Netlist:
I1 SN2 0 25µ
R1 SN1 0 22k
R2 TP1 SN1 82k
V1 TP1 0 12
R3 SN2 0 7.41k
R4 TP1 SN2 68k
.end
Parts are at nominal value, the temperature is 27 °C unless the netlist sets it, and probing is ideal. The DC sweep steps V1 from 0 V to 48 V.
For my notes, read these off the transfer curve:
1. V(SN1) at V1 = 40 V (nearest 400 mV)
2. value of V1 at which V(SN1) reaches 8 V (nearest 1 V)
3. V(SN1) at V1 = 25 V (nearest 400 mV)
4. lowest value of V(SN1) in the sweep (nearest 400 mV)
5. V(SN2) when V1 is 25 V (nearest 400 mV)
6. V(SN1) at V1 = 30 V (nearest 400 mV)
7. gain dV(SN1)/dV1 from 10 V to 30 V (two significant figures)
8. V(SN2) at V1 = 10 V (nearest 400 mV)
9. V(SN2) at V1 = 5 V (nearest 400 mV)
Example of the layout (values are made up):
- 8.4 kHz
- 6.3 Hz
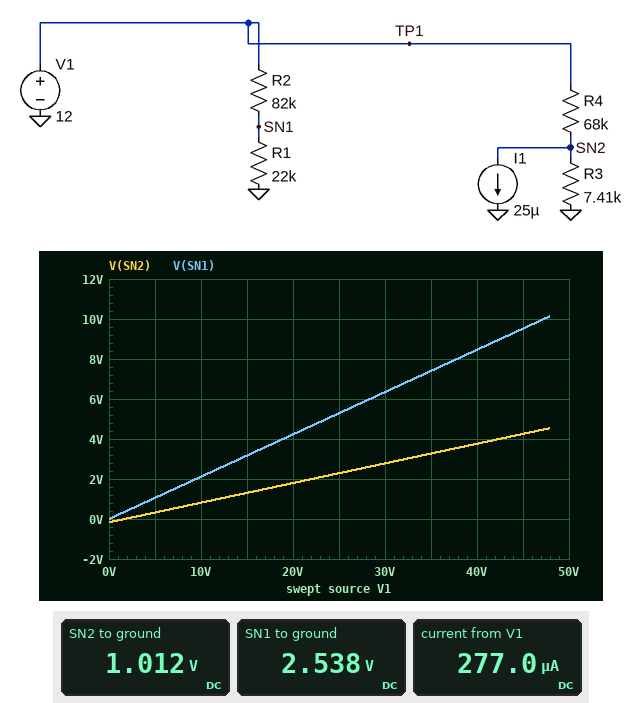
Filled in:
- 8.4 V
- 38 V
- 5.2 V
- 0 V
- 2.4 V
- 6.4 V
- 0.21 V/V
- 800 mV
- 400 mV
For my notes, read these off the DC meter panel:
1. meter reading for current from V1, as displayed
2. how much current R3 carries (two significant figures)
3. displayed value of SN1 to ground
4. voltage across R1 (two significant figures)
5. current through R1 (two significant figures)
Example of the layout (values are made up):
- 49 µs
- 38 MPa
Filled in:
- 277.0 µA
- 140 µA
- 2.538 V
- 2.5 V
- 120 µA
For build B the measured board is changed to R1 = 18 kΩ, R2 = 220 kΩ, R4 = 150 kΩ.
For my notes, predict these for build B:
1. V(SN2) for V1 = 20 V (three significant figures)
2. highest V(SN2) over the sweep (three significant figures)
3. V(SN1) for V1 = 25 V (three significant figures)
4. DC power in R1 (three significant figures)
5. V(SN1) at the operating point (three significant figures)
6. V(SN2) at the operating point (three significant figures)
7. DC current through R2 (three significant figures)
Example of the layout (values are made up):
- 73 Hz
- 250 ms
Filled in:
- 765 mV
- 2.08 V
- 1.89 V
- 45.8 µW
- 908 mV
- 388 mV
- 50.4 µA
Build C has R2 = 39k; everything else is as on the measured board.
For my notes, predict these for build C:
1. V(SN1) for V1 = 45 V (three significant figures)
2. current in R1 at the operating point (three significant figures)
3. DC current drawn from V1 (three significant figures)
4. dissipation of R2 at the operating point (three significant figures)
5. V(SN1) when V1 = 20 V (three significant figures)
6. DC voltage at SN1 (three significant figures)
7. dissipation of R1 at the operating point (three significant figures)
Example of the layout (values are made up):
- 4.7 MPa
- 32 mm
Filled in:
- 16.2 V
- 197 µA
- 358 µA
- 1.51 mW
- 7.21 V
- 4.33 V
- 851 µW
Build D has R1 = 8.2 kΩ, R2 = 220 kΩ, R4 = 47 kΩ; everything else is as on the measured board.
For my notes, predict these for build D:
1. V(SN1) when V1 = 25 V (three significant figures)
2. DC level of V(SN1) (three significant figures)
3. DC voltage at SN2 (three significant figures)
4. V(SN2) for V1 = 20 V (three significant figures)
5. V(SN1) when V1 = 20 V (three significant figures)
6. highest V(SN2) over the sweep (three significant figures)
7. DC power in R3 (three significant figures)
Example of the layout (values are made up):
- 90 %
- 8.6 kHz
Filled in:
- 898 mV
- 431 mV
- 1.47 V
- 2.56 V
- 719 mV
- 6.38 V
- 293 µW
